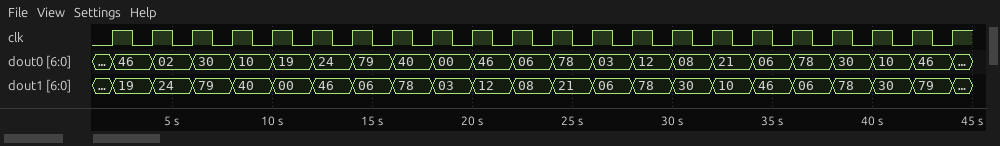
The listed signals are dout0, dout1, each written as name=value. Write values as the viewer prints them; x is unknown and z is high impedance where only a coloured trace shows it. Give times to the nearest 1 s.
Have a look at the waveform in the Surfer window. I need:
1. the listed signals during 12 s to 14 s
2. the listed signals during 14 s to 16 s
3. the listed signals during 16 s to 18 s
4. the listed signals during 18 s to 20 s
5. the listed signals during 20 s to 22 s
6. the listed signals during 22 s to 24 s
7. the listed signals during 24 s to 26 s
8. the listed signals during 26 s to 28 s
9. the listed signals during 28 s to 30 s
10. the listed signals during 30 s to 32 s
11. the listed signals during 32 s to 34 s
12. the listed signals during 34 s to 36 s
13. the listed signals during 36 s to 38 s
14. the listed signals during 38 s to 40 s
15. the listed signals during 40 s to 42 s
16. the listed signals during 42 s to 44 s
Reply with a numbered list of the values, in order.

1. dout0=24, dout1=46
2. dout0=79, dout1=06
3. dout0=40, dout1=78
4. dout0=00, dout1=03
5. dout0=46, dout1=12
6. dout0=06, dout1=08
7. dout0=78, dout1=21
8. dout0=03, dout1=06
9. dout0=12, dout1=78
10. dout0=08, dout1=30
11. dout0=21, dout1=10
12. dout0=06, dout1=46
13. dout0=78, dout1=06
14. dout0=30, dout1=78
15. dout0=10, dout1=30
16. dout0=46, dout1=79
